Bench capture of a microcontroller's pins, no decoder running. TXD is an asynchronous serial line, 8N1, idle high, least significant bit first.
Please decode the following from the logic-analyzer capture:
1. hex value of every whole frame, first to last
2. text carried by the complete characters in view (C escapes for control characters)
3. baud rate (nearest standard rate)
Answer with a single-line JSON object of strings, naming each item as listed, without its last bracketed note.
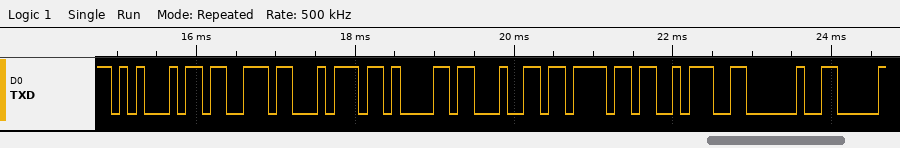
{"hex value of every whole frame, first to last": "0x45 0x73 0x74 0x61 0x64 0x6F 0x3A 0x20", "text carried by the complete characters in view": "\"Estado: \"", "baud rate": "9600 baud"}
